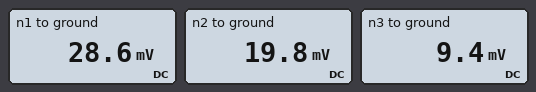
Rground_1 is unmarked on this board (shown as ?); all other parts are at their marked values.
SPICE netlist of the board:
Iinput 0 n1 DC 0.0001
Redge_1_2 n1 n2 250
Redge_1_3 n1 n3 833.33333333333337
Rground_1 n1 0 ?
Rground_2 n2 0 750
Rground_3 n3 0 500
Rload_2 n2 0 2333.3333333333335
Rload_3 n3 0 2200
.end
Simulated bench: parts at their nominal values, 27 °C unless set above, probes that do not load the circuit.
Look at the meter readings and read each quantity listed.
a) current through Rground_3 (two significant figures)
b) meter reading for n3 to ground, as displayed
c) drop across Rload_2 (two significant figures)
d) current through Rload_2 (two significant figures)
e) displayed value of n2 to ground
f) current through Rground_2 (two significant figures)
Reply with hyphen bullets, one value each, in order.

- 19 µA
- 9.4 mV
- 20 mV
- 8.5 µA
- 19.8 mV
- 26 µA
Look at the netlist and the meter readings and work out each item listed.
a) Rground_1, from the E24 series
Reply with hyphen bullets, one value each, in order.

- 680 Ω
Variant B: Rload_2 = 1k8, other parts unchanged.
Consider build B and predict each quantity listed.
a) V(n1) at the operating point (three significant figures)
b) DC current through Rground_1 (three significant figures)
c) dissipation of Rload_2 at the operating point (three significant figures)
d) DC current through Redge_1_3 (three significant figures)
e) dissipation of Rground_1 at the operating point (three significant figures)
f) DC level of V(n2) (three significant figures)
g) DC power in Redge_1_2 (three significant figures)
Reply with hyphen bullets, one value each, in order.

- 28.1 mV
- 41.3 µA
- 202 nW
- 22.6 µA
- 1.16 µW
- 19.1 mV
- 325 nW
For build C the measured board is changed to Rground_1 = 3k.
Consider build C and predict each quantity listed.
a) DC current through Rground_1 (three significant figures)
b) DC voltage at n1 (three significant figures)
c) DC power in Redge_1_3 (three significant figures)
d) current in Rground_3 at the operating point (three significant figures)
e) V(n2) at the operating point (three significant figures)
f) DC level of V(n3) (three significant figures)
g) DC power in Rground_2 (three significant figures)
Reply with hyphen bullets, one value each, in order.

- 14.1 µA
- 42.3 mV
- 970 nW
- 27.8 µA
- 29.4 mV
- 13.9 mV
- 1.15 µW
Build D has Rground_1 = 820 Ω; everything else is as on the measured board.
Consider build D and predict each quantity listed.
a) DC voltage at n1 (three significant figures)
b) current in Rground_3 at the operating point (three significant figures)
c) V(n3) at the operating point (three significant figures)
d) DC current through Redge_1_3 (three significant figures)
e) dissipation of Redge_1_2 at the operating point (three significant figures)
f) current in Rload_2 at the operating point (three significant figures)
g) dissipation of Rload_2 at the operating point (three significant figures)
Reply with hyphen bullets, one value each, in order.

- 30.8 mV
- 20.2 µA
- 10.1 mV
- 24.8 µA
- 354 nW
- 9.16 µA
- 196 nW
